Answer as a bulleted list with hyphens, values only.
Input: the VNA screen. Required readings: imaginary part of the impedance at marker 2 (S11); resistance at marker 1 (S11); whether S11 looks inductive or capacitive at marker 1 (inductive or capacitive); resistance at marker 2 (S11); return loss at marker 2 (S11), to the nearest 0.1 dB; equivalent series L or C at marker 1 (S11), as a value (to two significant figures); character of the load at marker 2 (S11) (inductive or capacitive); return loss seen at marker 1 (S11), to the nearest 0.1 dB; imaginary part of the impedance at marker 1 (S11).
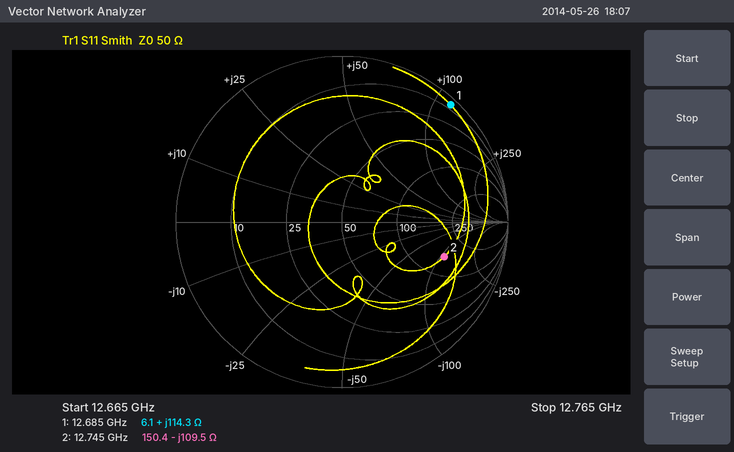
- -109.5 Ω
- 6.1 Ω
- inductive
- 150.4 Ω
- 3.7 dB
- 1.4 nH
- capacitive
- 0.3 dB
- +114.3 Ω
